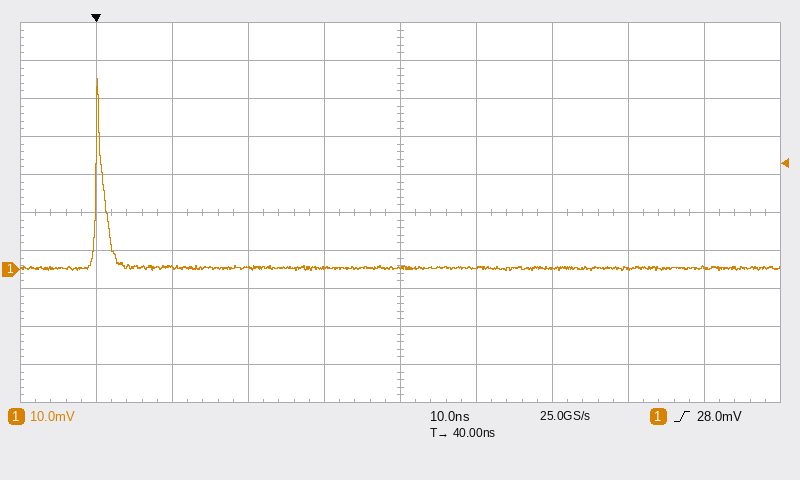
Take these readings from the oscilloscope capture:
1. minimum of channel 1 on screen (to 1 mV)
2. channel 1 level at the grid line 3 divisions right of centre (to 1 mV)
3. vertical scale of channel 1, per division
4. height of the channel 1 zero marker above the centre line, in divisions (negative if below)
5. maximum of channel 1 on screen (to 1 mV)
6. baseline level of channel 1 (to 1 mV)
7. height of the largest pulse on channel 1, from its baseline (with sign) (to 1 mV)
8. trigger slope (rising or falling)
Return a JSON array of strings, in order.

["0 mV", "0 mV", "10 mV", "-1.5 div", "50 mV", "0 mV", "+50 mV", "rising"]
